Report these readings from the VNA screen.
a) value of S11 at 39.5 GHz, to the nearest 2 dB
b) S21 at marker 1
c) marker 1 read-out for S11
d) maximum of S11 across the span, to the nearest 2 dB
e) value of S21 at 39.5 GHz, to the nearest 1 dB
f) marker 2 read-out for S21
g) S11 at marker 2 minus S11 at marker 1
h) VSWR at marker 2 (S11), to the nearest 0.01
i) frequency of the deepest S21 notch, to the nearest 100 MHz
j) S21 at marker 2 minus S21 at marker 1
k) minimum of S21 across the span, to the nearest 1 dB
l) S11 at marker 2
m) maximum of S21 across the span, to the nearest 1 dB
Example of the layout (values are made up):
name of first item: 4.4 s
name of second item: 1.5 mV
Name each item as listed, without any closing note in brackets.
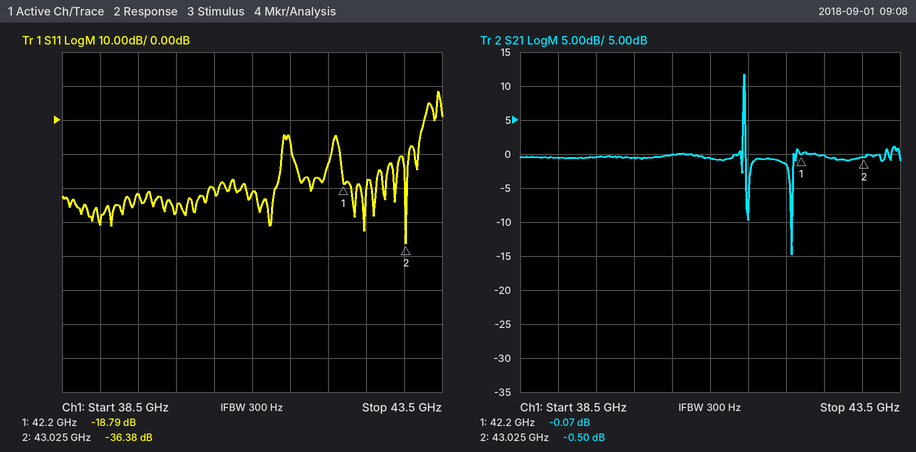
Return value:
value of S11 at 39.5 GHz, to the nearest 2 dB: -22 dB
S21 at marker 1: -0.07 dB
marker 1 read-out for S11: -18.79 dB
maximum of S11 across the span, to the nearest 2 dB: 8 dB
value of S21 at 39.5 GHz, to the nearest 1 dB: 0 dB
marker 2 read-out for S21: -0.50 dB
S11 at marker 2 minus S11 at marker 1: -17.59 dB
VSWR at marker 2 (S11), to the nearest 0.01: 1.03
frequency of the deepest S21 notch, to the nearest 100 MHz: 42.1 GHz
S21 at marker 2 minus S21 at marker 1: -0.43 dB
minimum of S21 across the span, to the nearest 1 dB: -15 dB
S11 at marker 2: -36.38 dB
maximum of S21 across the span, to the nearest 1 dB: 12 dB
